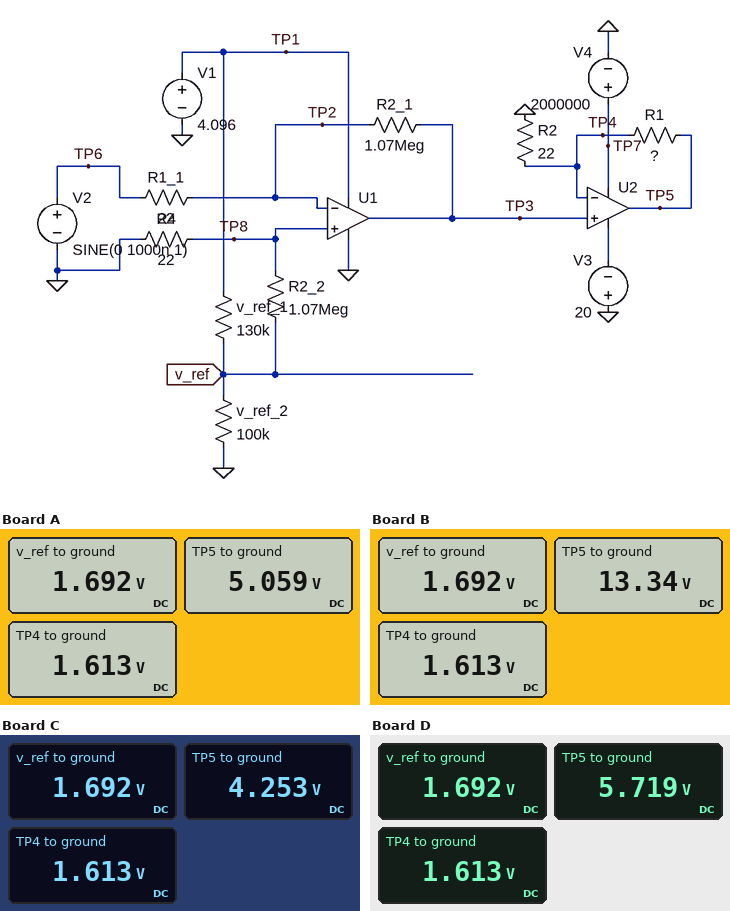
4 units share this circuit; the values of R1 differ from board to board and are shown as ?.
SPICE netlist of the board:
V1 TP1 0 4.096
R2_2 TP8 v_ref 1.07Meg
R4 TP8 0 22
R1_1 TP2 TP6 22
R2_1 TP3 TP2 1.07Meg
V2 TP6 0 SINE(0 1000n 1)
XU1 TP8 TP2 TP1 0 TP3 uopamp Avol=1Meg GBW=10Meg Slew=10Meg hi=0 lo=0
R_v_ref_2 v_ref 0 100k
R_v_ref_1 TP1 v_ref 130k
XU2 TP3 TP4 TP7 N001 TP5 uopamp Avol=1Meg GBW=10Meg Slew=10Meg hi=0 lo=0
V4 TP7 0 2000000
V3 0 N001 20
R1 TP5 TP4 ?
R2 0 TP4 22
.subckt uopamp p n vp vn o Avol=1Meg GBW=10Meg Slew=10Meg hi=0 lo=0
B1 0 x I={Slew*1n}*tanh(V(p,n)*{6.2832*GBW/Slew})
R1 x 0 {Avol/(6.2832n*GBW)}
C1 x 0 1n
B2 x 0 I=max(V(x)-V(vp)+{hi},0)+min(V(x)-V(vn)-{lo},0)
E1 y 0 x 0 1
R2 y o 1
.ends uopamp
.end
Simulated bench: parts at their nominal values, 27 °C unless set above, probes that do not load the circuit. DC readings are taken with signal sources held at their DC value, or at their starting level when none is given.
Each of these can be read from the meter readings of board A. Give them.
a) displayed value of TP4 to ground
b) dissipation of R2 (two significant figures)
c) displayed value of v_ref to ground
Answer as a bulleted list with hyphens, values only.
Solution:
- 1.613 V
- 120 mW
- 1.692 V
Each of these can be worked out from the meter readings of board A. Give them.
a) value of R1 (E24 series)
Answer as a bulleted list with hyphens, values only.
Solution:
- 47 Ω
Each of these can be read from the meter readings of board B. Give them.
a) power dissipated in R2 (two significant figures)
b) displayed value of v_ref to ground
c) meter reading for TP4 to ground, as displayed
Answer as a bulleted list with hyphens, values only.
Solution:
- 120 mW
- 1.692 V
- 1.613 V
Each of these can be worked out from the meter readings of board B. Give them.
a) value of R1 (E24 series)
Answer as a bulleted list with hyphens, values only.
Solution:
- 160 Ω
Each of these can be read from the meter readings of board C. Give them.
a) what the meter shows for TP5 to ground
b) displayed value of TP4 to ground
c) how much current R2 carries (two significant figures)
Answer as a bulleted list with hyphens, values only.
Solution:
- 4.253 V
- 1.613 V
- 73 mA
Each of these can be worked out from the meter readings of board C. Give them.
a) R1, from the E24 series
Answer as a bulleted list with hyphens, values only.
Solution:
- 36 Ω
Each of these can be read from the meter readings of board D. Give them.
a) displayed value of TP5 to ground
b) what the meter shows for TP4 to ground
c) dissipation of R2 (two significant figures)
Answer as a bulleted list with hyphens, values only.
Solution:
- 5.719 V
- 1.613 V
- 120 mW
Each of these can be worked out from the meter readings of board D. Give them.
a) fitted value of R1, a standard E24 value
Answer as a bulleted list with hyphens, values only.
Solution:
- 56 Ω
